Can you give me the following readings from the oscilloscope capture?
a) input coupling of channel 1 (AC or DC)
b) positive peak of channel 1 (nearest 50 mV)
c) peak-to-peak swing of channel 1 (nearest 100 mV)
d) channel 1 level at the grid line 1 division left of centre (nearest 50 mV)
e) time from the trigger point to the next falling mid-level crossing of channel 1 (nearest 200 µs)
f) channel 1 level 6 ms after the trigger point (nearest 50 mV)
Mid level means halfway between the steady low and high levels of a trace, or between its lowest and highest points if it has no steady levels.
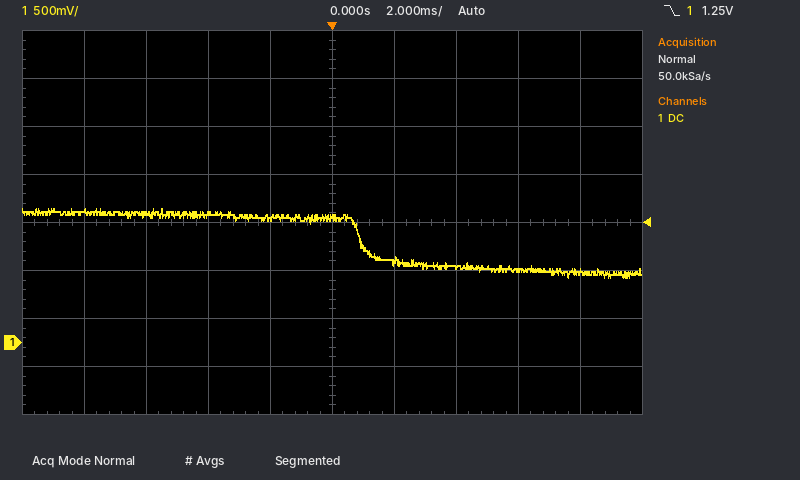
DC
1.40 V
700 mV
1.30 V
1.0 ms
750 mV
